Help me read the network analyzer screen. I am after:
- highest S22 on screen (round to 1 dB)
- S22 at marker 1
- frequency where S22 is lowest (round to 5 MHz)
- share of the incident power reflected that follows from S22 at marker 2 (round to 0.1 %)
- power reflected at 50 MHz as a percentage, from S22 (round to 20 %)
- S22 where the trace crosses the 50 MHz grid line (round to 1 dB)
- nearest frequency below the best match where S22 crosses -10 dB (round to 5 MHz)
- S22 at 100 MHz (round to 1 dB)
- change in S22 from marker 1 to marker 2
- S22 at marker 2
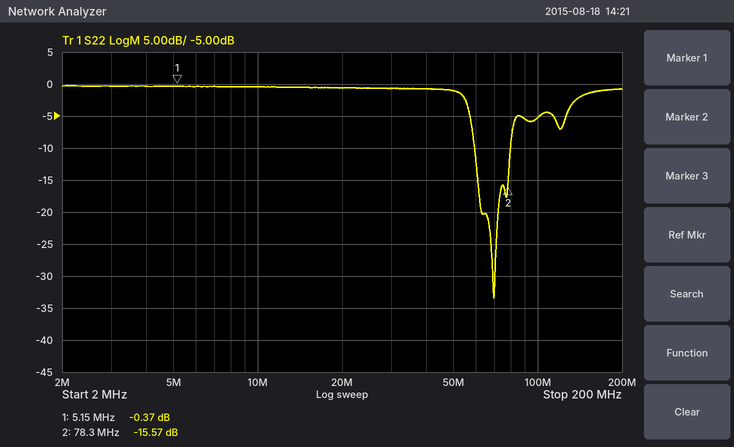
0 dB
-0.37 dB
70 MHz
2.8 %
80 %
-1 dB
60 MHz
-5 dB
-15.20 dB
-15.57 dB
